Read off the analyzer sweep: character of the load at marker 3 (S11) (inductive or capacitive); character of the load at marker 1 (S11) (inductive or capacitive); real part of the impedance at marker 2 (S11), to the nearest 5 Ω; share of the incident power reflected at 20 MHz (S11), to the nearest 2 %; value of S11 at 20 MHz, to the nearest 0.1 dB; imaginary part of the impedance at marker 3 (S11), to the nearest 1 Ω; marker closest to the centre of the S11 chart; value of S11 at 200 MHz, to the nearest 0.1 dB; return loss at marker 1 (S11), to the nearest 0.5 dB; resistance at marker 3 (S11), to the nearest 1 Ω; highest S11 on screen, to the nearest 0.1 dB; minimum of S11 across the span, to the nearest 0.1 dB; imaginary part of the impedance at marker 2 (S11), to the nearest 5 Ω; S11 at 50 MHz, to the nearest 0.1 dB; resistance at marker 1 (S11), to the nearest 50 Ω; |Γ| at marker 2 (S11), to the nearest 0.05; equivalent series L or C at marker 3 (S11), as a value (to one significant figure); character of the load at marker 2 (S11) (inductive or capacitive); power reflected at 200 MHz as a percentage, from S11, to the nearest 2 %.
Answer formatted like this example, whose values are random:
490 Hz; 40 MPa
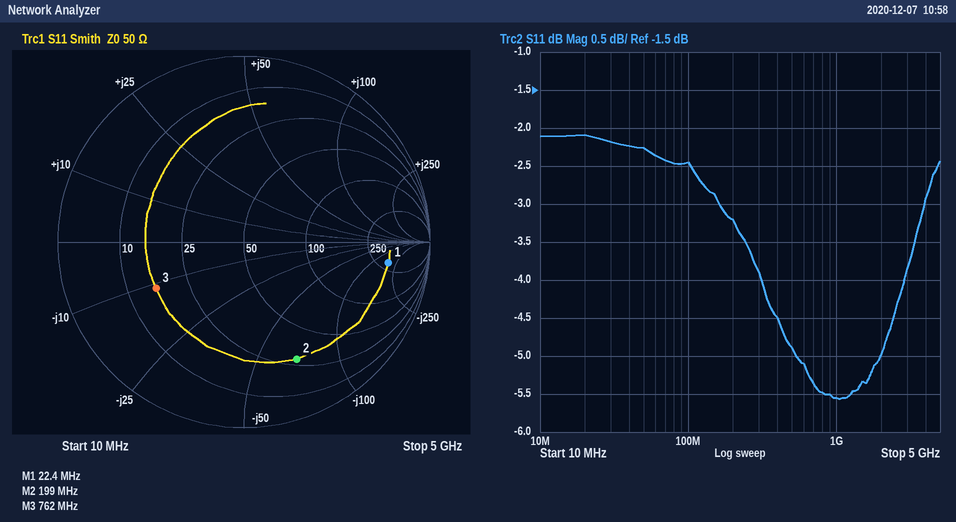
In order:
capacitive; capacitive; 30 Ω; 62 %; -2.1 dB; -11 Ω; marker 3; -3.2 dB; 2.0 dB; 16 Ω; -2.1 dB; -5.6 dB; -70 Ω; -2.3 dB; 300 Ω; 0.70; 20 pF; capacitive; 48 %
